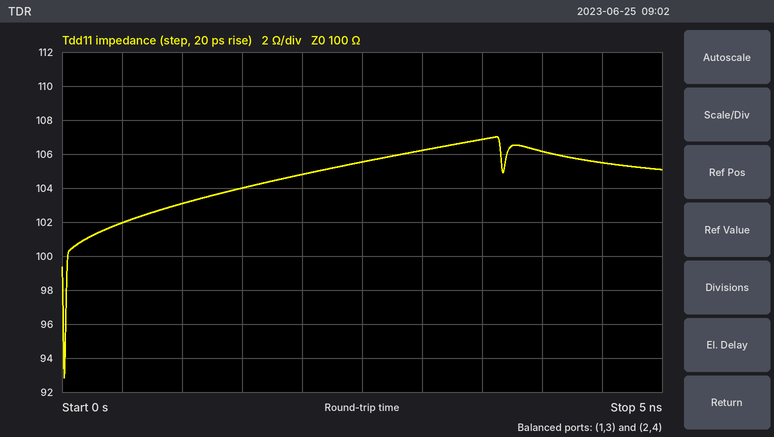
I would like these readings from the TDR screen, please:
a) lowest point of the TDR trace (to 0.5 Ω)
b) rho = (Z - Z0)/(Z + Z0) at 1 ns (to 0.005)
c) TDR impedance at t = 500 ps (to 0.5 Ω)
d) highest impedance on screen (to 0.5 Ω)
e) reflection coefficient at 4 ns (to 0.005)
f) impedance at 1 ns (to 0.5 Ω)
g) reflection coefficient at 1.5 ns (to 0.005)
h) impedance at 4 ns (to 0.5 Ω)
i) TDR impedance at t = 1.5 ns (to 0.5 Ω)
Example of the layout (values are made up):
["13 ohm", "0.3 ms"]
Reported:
["93.0 Ω", "+0.015", "102.0 Ω", "107.0 Ω", "+0.030", "103.0 Ω", "+0.020", "106.0 Ω", "104.0 Ω"]
